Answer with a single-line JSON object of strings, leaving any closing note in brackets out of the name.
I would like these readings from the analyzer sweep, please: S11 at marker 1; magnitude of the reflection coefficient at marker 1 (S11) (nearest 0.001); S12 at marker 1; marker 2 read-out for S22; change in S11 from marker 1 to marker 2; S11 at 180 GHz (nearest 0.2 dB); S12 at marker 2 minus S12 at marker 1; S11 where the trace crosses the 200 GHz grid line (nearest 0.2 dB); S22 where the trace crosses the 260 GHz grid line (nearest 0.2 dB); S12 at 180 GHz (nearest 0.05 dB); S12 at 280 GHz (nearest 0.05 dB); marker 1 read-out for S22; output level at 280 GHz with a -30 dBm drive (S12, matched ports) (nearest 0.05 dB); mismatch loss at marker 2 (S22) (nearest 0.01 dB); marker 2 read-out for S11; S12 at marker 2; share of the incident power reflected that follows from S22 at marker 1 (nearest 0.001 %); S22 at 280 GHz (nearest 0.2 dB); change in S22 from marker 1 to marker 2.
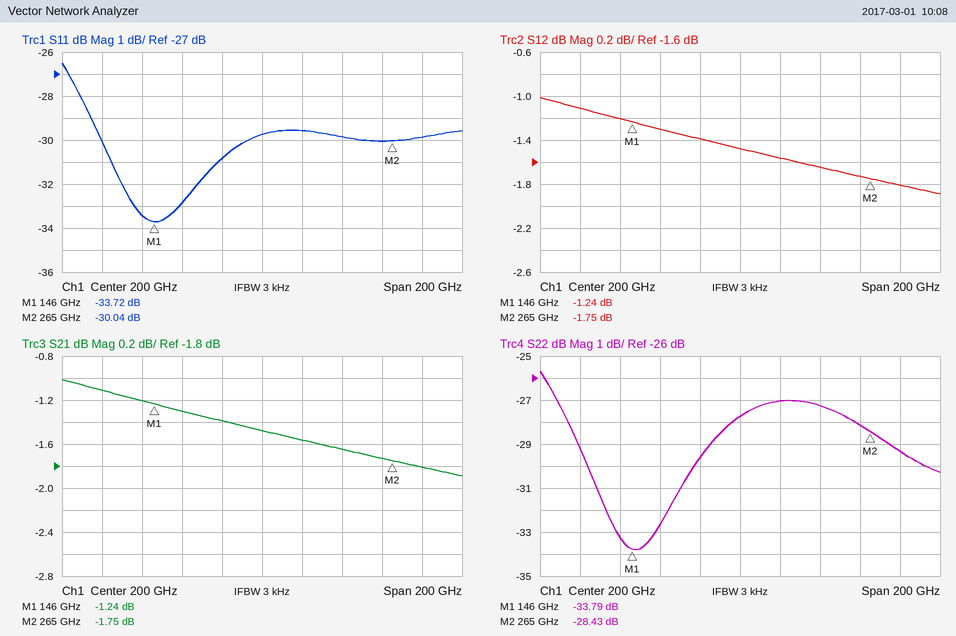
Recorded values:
{"S11 at marker 1": "-33.72 dB", "magnitude of the reflection coefficient at marker 1 (S11)": "0.021", "S12 at marker 1": "-1.24 dB", "marker 2 read-out for S22": "-28.43 dB", "change in S11 from marker 1 to marker 2": "3.68 dB", "S11 at 180 GHz": "-30.8 dB", "S12 at marker 2 minus S12 at marker 1": "-0.51 dB", "S11 where the trace crosses the 200 GHz grid line": "-29.8 dB", "S22 where the trace crosses the 260 GHz grid line": "-28.2 dB", "S12 at 180 GHz": "-1.40 dB", "S12 at 280 GHz": "-1.80 dB", "marker 1 read-out for S22": "-33.79 dB", "output level at 280 GHz with a -30 dBm drive (S12, matched ports)": "-31.80 dBm", "mismatch loss at marker 2 (S22)": "0.01 dB", "marker 2 read-out for S11": "-30.04 dB", "S12 at marker 2": "-1.75 dB", "share of the incident power reflected that follows from S22 at marker 1": "0.042 %", "S22 at 280 GHz": "-29.4 dB", "change in S22 from marker 1 to marker 2": "5.36 dB"}
